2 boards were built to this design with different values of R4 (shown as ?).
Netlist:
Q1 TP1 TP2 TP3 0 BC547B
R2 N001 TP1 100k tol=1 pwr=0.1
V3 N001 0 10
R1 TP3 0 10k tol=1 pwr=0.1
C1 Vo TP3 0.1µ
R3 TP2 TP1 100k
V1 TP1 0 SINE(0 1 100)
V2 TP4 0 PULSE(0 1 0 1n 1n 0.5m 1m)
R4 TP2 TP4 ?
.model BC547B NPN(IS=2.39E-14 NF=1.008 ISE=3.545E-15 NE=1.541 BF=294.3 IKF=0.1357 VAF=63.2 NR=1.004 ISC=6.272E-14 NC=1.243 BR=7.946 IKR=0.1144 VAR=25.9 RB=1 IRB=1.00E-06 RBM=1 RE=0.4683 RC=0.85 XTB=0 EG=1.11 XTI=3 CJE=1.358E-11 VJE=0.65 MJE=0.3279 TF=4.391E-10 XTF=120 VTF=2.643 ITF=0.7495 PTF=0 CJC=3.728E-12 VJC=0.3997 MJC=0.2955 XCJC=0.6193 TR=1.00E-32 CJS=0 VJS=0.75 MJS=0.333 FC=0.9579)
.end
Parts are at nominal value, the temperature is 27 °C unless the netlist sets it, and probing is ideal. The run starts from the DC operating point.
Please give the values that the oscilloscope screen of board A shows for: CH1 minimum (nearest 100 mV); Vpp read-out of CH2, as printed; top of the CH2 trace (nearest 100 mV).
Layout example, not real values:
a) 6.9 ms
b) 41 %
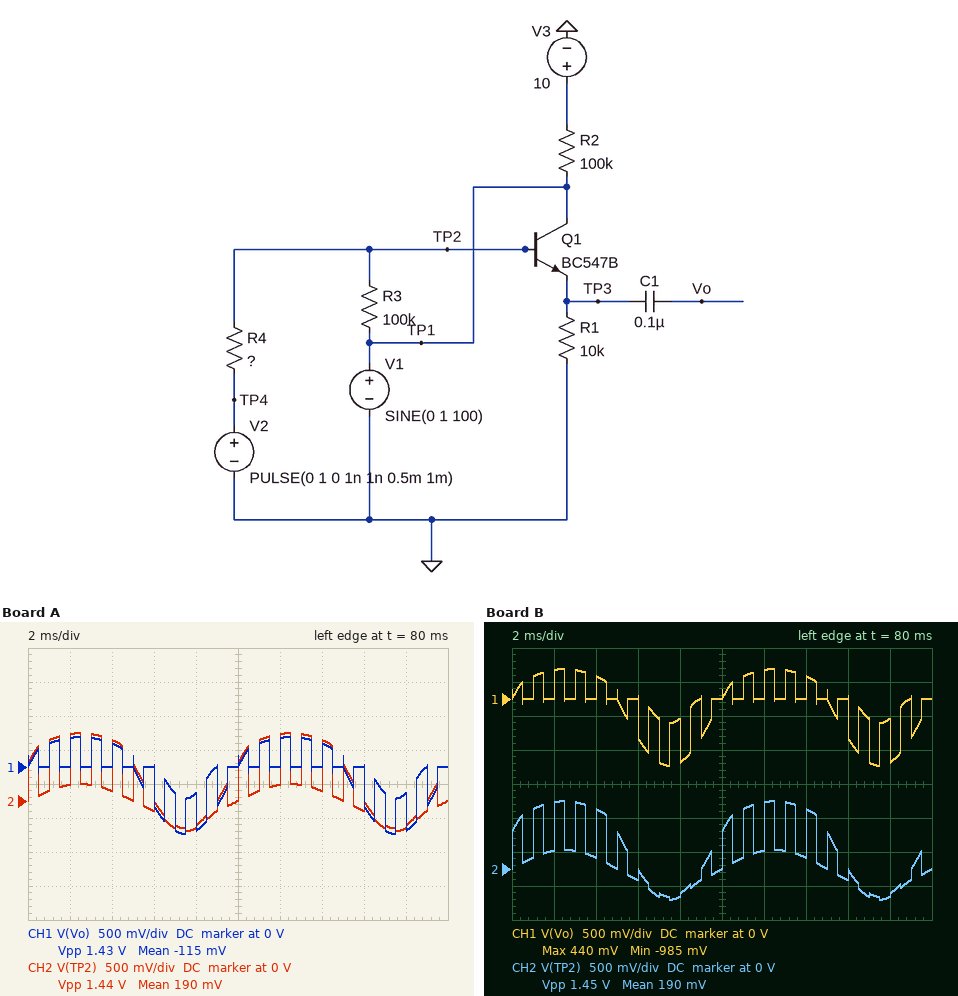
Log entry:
a) -1.0 V
b) 1.44 V
c) 1.0 V
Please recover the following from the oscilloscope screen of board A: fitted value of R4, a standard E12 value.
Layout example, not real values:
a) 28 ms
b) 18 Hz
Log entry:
a) 33 kΩ
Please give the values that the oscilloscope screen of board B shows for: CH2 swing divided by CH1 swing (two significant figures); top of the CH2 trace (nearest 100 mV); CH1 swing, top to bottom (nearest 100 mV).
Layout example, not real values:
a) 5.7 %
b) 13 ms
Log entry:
a) 1.0
b) 1.0 V
c) 1.4 V
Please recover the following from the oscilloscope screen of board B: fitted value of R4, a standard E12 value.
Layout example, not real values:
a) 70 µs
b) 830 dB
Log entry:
a) 39 kΩ
